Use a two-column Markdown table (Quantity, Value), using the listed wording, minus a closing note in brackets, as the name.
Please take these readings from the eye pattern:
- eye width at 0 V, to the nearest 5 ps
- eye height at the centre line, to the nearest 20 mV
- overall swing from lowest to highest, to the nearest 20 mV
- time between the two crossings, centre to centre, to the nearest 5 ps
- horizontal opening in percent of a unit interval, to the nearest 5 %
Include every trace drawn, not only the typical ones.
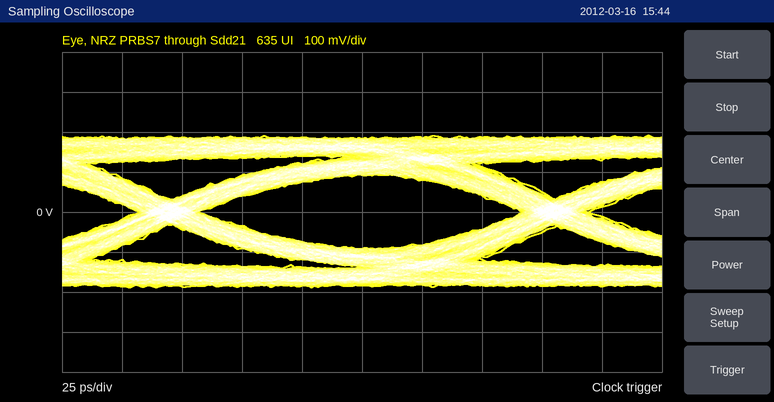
| Quantity | Value |
|---|---|
| eye width at 0 V, to the nearest 5 ps | 135 ps |
| eye height at the centre line, to the nearest 20 mV | 180 mV |
| overall swing from lowest to highest, to the nearest 20 mV | 380 mV |
| time between the two crossings, centre to centre, to the nearest 5 ps | 160 ps |
| horizontal opening in percent of a unit interval, to the nearest 5 % | 85 % |
